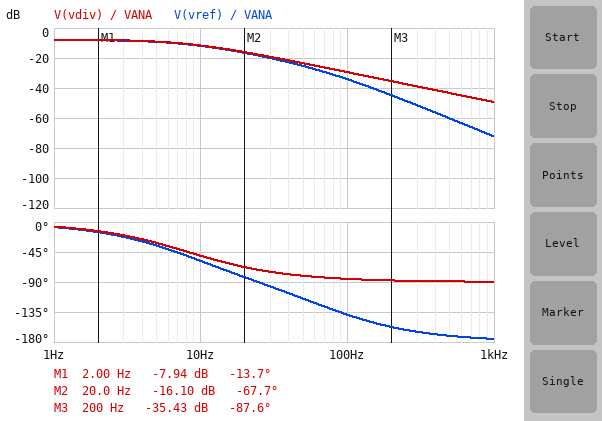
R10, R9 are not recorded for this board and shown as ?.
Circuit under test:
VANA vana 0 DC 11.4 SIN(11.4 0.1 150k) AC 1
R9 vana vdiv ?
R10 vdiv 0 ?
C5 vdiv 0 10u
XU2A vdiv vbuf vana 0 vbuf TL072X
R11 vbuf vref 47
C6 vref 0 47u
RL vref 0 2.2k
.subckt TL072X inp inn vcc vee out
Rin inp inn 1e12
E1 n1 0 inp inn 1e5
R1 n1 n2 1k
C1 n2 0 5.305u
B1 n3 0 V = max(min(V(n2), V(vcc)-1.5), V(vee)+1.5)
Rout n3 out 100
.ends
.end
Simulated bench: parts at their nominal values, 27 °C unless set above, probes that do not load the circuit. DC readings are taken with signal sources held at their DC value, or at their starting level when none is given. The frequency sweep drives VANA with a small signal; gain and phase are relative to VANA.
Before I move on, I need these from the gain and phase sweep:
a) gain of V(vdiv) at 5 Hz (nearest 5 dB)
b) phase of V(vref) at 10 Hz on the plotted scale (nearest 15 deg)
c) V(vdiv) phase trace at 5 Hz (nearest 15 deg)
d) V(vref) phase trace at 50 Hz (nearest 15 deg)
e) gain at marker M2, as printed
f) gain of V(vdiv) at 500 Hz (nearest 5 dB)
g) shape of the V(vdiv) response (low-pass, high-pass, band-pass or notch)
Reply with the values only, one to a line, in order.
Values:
-10 dB
-60 deg
-30 deg
-120 deg
-16.10 dB
-45 dB
low-pass
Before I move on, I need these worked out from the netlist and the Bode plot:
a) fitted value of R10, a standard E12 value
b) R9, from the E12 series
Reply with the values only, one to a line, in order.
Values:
3.3 kΩ
4.7 kΩ
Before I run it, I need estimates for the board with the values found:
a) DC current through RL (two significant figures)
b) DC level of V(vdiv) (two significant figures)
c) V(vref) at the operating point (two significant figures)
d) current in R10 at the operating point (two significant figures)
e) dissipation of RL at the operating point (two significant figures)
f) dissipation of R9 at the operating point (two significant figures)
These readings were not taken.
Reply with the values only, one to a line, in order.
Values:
2.1 mA
4.7 V
4.6 V
1.4 mA
9.6 mW
9.5 mW
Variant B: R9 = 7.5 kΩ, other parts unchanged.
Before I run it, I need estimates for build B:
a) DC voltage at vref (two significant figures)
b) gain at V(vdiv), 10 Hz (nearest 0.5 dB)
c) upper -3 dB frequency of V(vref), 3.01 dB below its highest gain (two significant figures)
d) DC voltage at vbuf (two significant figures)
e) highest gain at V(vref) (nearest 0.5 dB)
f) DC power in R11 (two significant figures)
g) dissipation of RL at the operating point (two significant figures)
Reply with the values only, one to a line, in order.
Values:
3.4 V
-15.0 dB
6.9 Hz
3.5 V
-10.5 dB
110 µW
5.3 mW
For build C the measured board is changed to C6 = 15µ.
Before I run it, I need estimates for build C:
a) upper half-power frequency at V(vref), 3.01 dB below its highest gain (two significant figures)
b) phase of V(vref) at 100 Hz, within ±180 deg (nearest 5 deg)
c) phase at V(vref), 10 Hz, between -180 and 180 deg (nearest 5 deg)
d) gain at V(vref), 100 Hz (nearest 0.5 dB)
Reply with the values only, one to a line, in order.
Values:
8.2 Hz
-110 deg
-55 deg
-30.5 dB
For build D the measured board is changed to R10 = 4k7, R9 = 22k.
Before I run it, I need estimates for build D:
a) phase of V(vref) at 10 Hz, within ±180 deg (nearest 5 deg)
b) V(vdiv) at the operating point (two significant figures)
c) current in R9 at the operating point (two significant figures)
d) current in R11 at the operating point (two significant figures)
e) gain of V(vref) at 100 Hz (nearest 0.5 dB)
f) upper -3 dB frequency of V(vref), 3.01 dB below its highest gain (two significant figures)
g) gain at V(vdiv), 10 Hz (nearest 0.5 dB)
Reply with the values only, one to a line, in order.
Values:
-75 deg
2.0 V
430 µA
890 µA
-47.5 dB
4.1 Hz
-23.5 dB
